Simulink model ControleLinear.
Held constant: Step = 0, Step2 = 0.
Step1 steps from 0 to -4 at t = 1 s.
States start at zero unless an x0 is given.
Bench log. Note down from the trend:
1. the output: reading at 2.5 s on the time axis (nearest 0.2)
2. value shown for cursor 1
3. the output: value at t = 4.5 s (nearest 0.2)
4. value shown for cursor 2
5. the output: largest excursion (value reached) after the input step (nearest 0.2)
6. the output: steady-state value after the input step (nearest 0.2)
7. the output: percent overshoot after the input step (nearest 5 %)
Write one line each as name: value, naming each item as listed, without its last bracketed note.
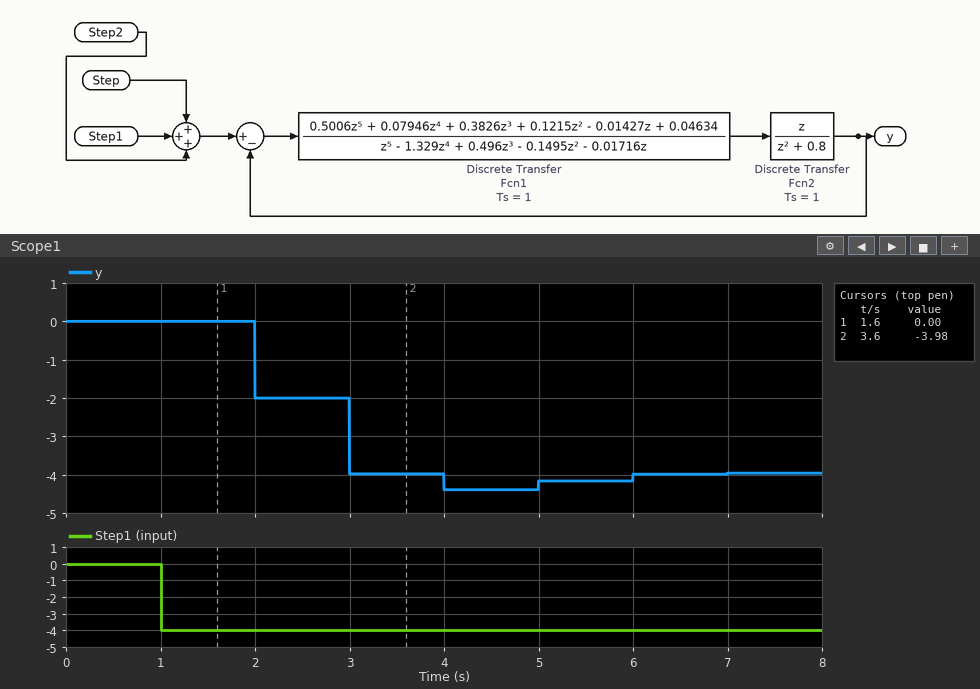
the output: reading at 2.5 s on the time axis: -2.0
value shown for cursor 1: 0.00
the output: value at t = 4.5 s: -4.4
value shown for cursor 2: -3.98
the output: largest excursion (value reached) after the input step: -4.4
the output: steady-state value after the input step: -4.0
the output: percent overshoot after the input step: 10 %
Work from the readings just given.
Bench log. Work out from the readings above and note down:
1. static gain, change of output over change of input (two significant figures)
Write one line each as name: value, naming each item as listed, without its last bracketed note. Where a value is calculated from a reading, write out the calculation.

static gain, change of output over change of input: (-4 - 0) / (-4 - 0) = 1.0
